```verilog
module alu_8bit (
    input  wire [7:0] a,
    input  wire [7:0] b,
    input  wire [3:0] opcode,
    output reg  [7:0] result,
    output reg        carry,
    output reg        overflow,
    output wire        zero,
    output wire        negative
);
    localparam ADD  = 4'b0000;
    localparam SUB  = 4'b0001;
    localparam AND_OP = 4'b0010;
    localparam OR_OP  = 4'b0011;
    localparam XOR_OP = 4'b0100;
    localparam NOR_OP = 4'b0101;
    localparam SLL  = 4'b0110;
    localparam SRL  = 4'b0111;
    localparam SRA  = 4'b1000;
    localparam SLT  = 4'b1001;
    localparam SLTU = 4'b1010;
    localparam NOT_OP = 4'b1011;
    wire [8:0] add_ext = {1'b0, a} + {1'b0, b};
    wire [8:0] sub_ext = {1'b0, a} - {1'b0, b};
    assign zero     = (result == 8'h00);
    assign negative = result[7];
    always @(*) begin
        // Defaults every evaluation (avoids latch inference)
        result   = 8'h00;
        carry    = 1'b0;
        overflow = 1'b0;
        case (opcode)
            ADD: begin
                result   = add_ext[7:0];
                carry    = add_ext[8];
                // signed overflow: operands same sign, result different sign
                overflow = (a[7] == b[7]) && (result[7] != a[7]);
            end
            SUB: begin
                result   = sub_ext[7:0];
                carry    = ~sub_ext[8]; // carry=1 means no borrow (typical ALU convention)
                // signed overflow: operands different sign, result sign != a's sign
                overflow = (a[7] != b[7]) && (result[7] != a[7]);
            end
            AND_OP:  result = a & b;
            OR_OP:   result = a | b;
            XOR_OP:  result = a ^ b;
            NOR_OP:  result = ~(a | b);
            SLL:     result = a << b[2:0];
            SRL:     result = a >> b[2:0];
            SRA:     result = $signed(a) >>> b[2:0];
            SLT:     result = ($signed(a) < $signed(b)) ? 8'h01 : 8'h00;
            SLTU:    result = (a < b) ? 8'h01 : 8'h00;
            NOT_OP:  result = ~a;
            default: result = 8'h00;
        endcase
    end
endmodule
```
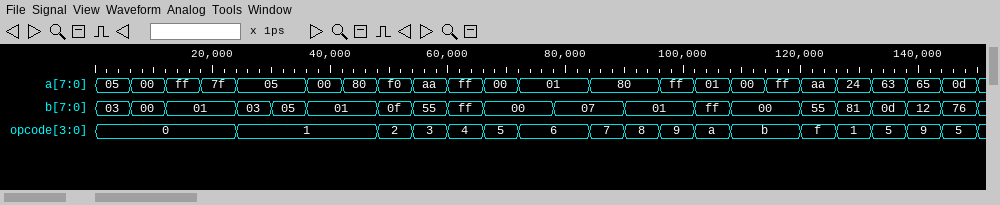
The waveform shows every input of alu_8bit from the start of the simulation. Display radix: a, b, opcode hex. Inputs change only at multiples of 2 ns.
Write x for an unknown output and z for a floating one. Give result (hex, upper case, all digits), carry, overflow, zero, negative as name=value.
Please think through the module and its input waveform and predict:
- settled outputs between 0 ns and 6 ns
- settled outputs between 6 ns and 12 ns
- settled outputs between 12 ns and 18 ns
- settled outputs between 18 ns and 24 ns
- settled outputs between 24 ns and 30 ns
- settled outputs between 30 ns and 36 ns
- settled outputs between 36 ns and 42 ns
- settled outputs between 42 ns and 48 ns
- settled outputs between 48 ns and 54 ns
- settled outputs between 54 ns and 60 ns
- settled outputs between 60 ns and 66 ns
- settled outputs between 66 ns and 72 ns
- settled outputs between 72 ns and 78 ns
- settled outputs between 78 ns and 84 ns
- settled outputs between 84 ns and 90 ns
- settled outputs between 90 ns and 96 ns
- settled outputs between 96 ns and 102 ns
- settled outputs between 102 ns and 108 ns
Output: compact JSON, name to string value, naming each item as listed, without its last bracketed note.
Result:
{"settled outputs between 0 ns and 6 ns": "result=08, carry=0, overflow=0, zero=0, negative=0", "settled outputs between 6 ns and 12 ns": "result=00, carry=0, overflow=0, zero=1, negative=0", "settled outputs between 12 ns and 18 ns": "result=00, carry=1, overflow=0, zero=1, negative=0", "settled outputs between 18 ns and 24 ns": "result=80, carry=0, overflow=1, zero=0, negative=1", "settled outputs between 24 ns and 30 ns": "result=02, carry=1, overflow=0, zero=0, negative=0", "settled outputs between 30 ns and 36 ns": "result=00, carry=1, overflow=0, zero=1, negative=0", "settled outputs between 36 ns and 42 ns": "result=FF, carry=0, overflow=0, zero=0, negative=1", "settled outputs between 42 ns and 48 ns": "result=7F, carry=1, overflow=1, zero=0, negative=0", "settled outputs between 48 ns and 54 ns": "result=00, carry=0, overflow=0, zero=1, negative=0", "settled outputs between 54 ns and 60 ns": "result=FF, carry=0, overflow=0, zero=0, negative=1", "settled outputs between 60 ns and 66 ns": "result=00, carry=0, overflow=0, zero=1, negative=0", "settled outputs between 66 ns and 72 ns": "result=FF, carry=0, overflow=0, zero=0, negative=1", "settled outputs between 72 ns and 78 ns": "result=01, carry=0, overflow=0, zero=0, negative=0", "settled outputs between 78 ns and 84 ns": "result=80, carry=0, overflow=0, zero=0, negative=1", "settled outputs between 84 ns and 90 ns": "result=01, carry=0, overflow=0, zero=0, negative=0", "settled outputs between 90 ns and 96 ns": "result=C0, carry=0, overflow=0, zero=0, negative=1", "settled outputs between 96 ns and 102 ns": "result=01, carry=0, overflow=0, zero=0, negative=0", "settled outputs between 102 ns and 108 ns": "result=01, carry=0, overflow=0, zero=0, negative=0"}
